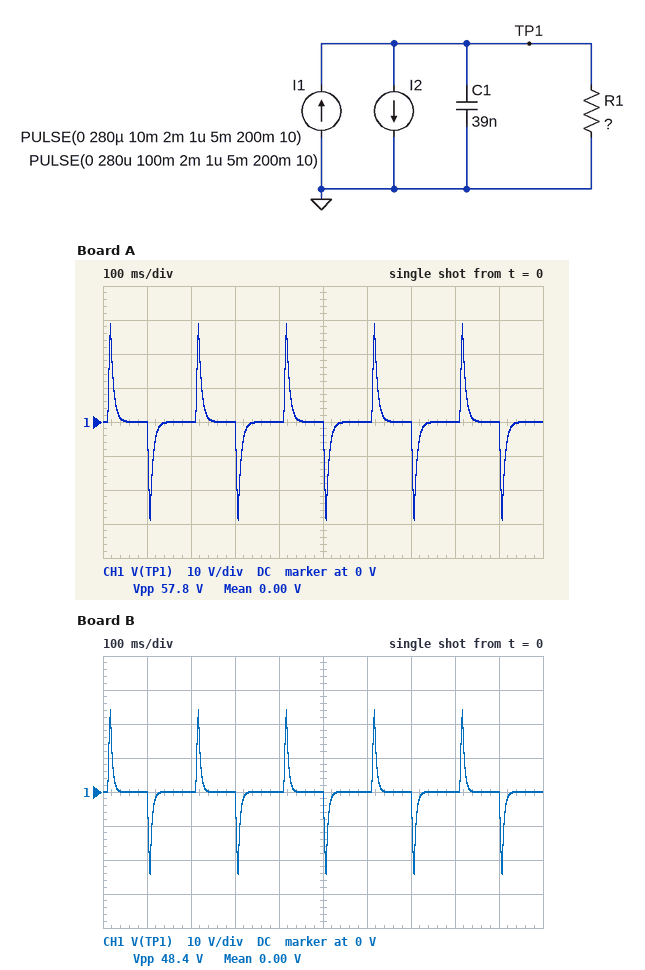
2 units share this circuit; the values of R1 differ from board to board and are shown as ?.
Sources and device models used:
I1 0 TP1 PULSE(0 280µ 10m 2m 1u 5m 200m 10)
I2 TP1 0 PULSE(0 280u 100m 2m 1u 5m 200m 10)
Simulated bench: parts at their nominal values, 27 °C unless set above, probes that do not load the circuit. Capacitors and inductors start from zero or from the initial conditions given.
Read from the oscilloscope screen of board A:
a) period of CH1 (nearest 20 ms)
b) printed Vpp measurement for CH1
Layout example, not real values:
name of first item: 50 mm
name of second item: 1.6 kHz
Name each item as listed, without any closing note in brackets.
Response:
period of CH1: 200 ms
printed Vpp measurement for CH1: 57.8 V
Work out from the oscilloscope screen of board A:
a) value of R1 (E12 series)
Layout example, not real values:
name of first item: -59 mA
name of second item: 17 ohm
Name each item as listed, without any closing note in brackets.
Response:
value of R1: 180 kΩ
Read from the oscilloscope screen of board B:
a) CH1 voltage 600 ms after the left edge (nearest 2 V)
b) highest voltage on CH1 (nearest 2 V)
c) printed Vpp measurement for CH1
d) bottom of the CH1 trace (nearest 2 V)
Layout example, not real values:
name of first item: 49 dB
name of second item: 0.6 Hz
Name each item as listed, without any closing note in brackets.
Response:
CH1 voltage 600 ms after the left edge: 0 V
highest voltage on CH1: 24 V
printed Vpp measurement for CH1: 48.4 V
bottom of the CH1 trace: -24 V
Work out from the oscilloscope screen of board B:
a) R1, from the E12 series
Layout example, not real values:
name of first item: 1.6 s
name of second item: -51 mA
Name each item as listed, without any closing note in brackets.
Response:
R1, from the E12 series: 120 kΩ
